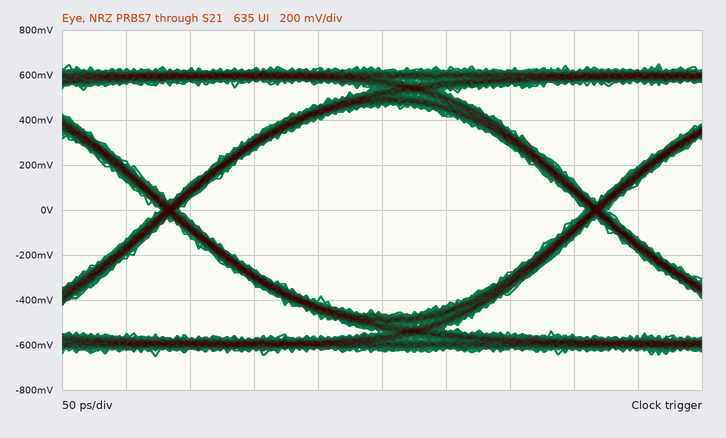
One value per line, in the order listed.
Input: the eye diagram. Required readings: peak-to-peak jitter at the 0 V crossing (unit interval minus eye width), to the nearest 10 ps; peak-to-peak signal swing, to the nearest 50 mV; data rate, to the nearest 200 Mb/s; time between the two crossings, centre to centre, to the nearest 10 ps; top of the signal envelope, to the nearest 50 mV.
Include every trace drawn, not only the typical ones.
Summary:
20 ps
1.30 V
3.0 Gb/s
330 ps
650 mV
